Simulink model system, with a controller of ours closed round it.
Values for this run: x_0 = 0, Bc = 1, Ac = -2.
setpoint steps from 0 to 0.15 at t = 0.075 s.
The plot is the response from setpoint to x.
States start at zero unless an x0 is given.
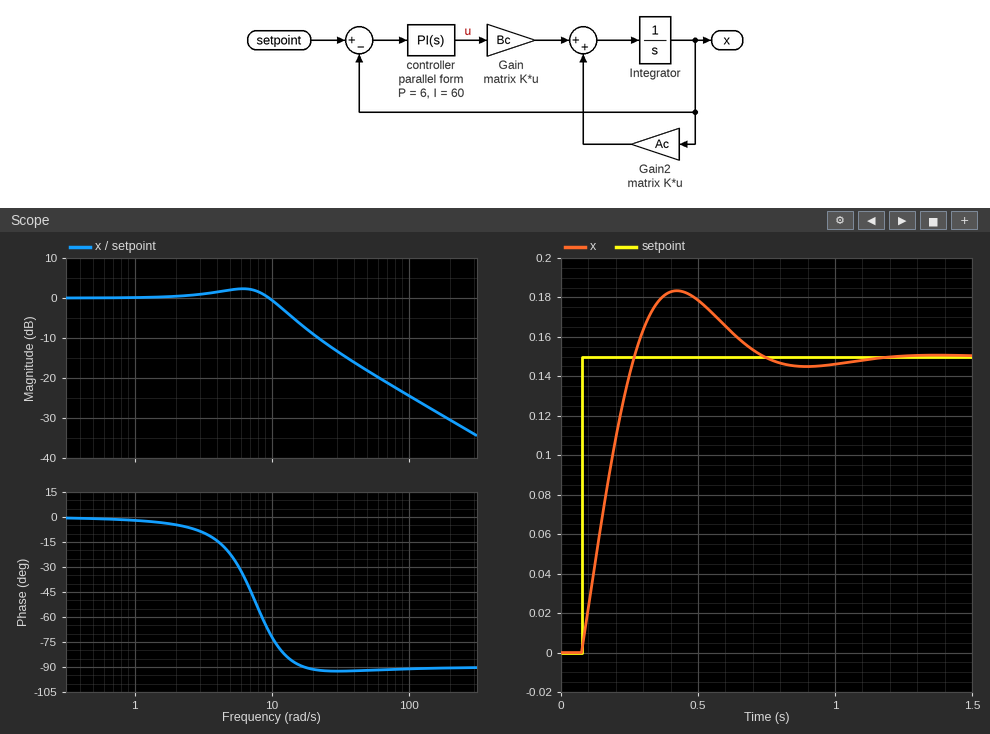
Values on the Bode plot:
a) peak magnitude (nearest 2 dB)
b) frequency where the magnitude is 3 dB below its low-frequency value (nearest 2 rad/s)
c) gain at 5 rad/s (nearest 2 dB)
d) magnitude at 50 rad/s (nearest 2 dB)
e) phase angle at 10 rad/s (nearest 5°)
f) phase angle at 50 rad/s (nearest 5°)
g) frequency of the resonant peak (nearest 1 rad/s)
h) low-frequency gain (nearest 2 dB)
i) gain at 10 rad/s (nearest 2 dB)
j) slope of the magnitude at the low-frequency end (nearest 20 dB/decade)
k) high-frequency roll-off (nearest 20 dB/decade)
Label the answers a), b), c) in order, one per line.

a) 2 dB
b) 12 rad/s
c) 2 dB
d) -18 dB
e) -70°
f) -90°
g) 6 rad/s
h) 0 dB
i) 0 dB
j) 0 dB/decade
k) -20 dB/decade
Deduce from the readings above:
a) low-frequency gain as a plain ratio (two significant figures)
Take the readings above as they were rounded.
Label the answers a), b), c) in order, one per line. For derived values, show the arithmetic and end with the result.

a) 10^(0 / 20) = 1.0
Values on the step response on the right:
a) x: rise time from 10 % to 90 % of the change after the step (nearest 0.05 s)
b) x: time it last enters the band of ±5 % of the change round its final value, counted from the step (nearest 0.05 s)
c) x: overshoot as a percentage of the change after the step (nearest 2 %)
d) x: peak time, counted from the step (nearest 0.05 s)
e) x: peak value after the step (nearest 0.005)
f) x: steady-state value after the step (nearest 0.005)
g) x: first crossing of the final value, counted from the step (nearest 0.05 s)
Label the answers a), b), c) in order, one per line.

a) 0.15 s
b) 0.60 s
c) 22 %
d) 0.35 s
e) 0.185
f) 0.150
g) 0.20 s
